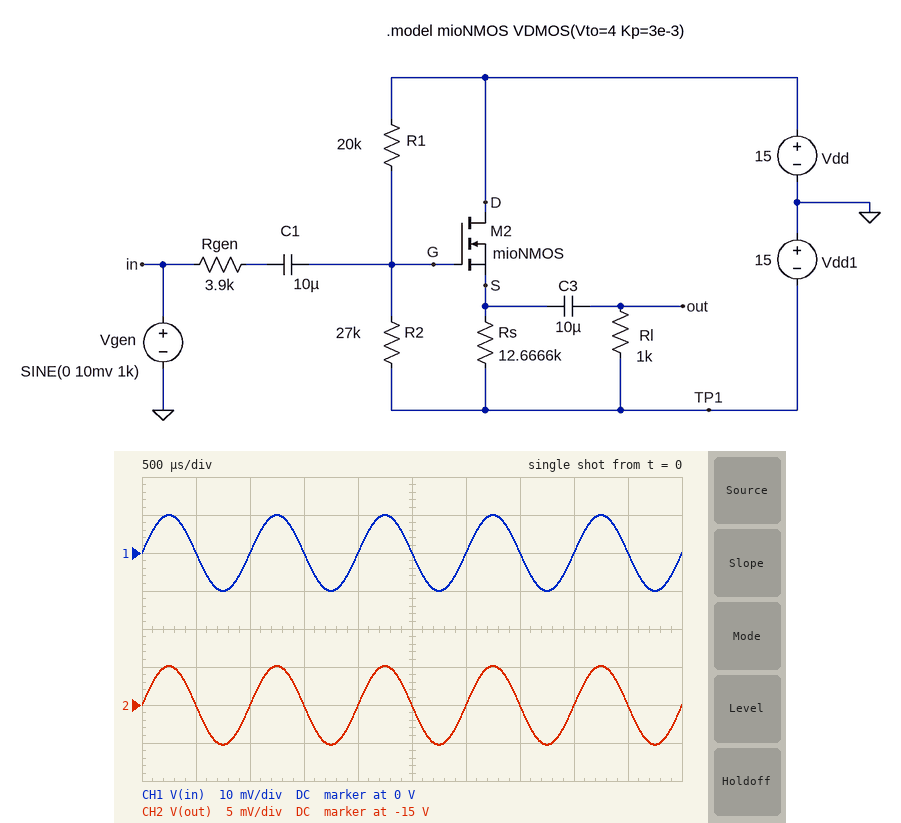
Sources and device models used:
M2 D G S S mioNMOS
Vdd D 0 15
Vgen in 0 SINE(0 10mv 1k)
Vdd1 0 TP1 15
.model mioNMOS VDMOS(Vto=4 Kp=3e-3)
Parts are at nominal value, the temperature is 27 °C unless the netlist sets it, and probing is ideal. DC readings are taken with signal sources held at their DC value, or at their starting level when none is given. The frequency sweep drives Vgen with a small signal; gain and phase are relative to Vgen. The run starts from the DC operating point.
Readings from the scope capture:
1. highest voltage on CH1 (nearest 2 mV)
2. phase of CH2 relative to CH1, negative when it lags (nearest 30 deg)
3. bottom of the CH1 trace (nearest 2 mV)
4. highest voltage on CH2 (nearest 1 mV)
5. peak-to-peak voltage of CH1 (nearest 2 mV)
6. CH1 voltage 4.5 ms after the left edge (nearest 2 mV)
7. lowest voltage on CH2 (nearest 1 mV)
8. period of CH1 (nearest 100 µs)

10 mV
0 deg
-10 mV
-14.995 V
20 mV
0 V
-15.005 V
1.0 ms
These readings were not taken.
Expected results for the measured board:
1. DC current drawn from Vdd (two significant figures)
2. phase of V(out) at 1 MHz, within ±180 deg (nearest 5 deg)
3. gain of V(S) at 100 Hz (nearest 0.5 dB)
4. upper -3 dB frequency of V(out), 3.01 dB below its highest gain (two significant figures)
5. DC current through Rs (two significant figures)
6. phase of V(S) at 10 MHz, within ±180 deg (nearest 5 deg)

1.6 mA
-50 deg
-5.5 dB
99 kHz
980 µA
-85 deg
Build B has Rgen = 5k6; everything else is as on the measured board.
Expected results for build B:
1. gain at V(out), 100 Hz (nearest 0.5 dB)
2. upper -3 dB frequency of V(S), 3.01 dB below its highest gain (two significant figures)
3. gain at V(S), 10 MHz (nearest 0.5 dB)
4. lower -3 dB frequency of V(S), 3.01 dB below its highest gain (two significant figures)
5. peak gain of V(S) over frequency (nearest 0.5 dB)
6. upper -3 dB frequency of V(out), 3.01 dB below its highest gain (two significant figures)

-6.5 dB
28 kHz
-36.5 dB
840 mHz
-4.0 dB
77 kHz
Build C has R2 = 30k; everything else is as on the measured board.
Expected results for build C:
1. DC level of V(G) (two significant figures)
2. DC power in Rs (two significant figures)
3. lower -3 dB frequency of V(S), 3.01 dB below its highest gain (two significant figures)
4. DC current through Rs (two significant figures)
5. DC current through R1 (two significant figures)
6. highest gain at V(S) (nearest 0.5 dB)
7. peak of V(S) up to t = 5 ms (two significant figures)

3.0 V
14 mW
900 mHz
1.0 mA
600 µA
-3.0 dB
-1.8 V
